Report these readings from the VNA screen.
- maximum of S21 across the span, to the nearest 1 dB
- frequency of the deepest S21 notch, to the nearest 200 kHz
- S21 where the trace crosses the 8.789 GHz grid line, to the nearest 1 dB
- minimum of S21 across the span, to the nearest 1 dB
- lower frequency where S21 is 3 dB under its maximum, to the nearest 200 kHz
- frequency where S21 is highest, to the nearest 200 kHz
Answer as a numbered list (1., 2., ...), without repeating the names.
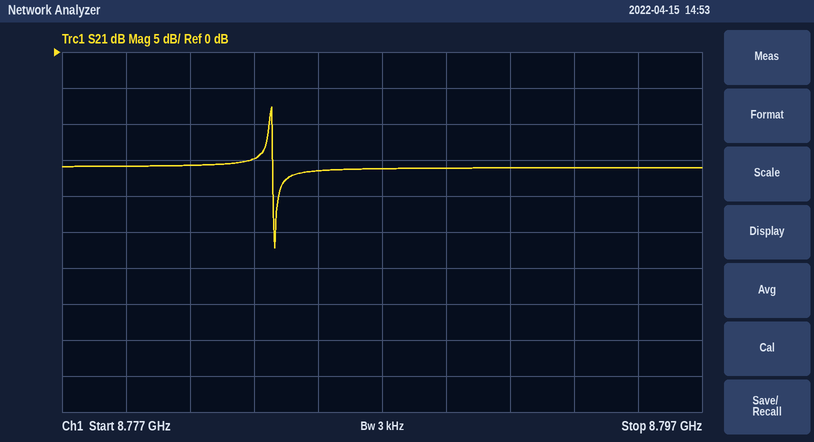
1. -8 dB
2. 8.7836 GHz
3. -16 dB
4. -27 dB
5. 8.7834 GHz
6. 8.7836 GHz
